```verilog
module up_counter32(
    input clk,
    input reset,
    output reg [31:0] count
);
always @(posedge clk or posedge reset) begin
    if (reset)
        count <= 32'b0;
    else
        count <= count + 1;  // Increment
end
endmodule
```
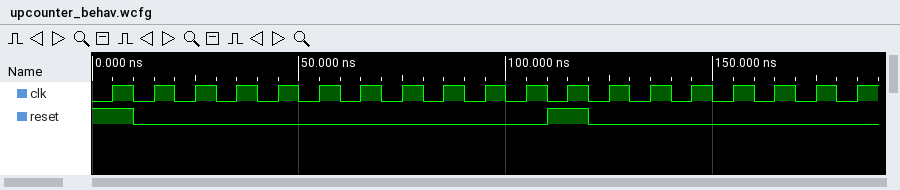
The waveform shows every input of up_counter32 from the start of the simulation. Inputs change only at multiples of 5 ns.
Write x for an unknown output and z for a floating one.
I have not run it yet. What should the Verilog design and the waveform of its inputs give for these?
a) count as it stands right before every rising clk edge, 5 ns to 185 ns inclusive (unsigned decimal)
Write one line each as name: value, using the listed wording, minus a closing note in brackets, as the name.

count as it stands right before every rising clk edge, 5 ns to 185 ns inclusive: 0, 0, 1, 2, 3, 4, 5, 6, 7, 8, 9, 0, 0, 1, 2, 3, 4, 5, 6
